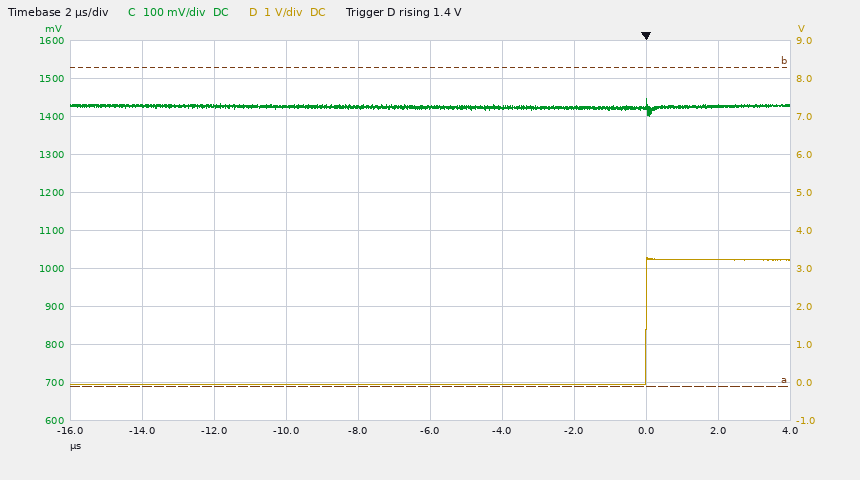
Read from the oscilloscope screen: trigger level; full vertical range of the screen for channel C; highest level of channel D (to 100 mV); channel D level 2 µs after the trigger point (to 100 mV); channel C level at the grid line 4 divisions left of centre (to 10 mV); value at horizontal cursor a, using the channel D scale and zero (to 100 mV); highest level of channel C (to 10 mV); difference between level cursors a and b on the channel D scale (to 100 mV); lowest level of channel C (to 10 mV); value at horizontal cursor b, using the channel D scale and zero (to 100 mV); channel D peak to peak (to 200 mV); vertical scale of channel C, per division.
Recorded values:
1.4 V
1 V
3.3 V
3.2 V
1.43 V
-100 mV
1.45 V
8.4 V
1.40 V
8.3 V
3.4 V
100 mV
